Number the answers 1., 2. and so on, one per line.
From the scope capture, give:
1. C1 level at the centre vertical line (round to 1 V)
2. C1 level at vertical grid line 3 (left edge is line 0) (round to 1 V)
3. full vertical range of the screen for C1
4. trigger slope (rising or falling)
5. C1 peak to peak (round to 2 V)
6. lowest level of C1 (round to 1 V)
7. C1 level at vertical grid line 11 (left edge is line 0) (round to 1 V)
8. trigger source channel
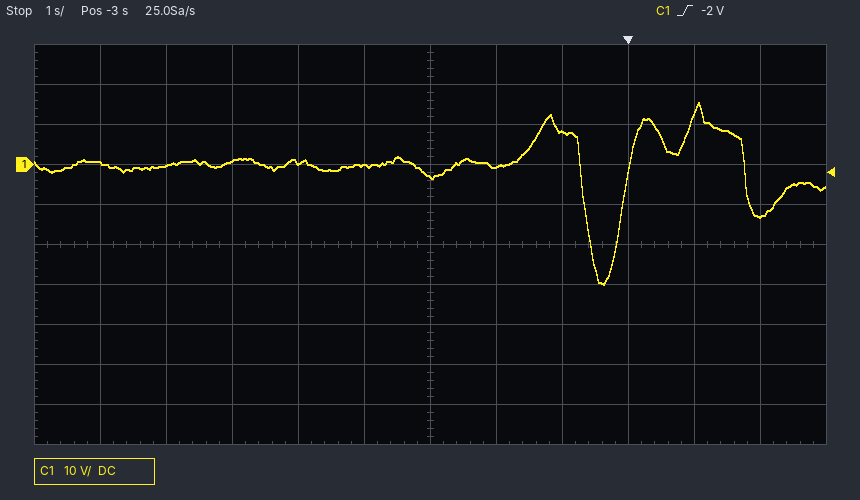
1. -3 V
2. 1 V
3. 100 V
4. rising
5. 46 V
6. -30 V
7. -13 V
8. C1
